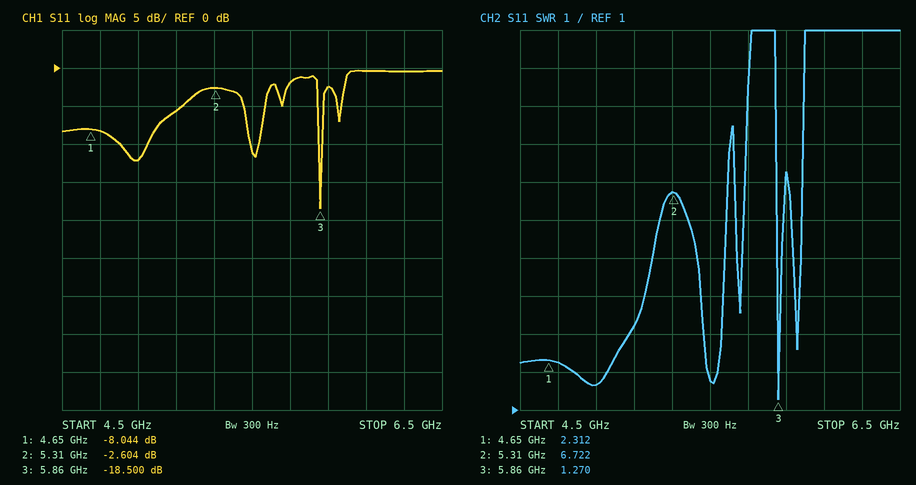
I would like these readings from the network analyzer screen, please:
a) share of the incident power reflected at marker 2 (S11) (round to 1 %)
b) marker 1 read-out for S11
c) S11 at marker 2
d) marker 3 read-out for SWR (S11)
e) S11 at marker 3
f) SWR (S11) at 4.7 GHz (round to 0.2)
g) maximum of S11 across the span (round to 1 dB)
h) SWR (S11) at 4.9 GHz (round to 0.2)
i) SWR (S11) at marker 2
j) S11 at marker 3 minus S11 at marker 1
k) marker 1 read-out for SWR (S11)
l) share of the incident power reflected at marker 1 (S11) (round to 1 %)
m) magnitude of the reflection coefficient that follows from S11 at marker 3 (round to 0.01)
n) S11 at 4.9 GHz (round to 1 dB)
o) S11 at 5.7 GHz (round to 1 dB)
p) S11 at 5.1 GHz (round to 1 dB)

55 %
-8.044 dB
-2.604 dB
1.270
-18.500 dB
2.2
0 dB
1.6
6.722
-10.456 dB
2.312
16 %
0.12
-12 dB
-2 dB
-6 dB
